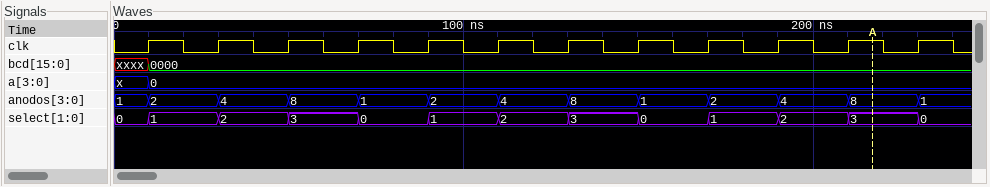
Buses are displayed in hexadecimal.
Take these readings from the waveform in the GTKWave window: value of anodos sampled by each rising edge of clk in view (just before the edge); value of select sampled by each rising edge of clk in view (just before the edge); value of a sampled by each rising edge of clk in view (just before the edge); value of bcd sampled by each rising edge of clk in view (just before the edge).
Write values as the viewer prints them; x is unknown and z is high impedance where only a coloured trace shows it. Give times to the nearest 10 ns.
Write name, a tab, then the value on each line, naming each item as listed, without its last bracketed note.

value of anodos sampled by each rising edge of clk in view	1, 2, 4, 8, 1, 2, 4, 8, 1, 2, 4, 8
value of select sampled by each rising edge of clk in view	0, 1, 2, 3, 0, 1, 2, 3, 0, 1, 2, 3
value of a sampled by each rising edge of clk in view	x, 0, 0, 0, 0, 0, 0, 0, 0, 0, 0, 0
value of bcd sampled by each rising edge of clk in view	xxxx, 0000, 0000, 0000, 0000, 0000, 0000, 0000, 0000, 0000, 0000, 0000
